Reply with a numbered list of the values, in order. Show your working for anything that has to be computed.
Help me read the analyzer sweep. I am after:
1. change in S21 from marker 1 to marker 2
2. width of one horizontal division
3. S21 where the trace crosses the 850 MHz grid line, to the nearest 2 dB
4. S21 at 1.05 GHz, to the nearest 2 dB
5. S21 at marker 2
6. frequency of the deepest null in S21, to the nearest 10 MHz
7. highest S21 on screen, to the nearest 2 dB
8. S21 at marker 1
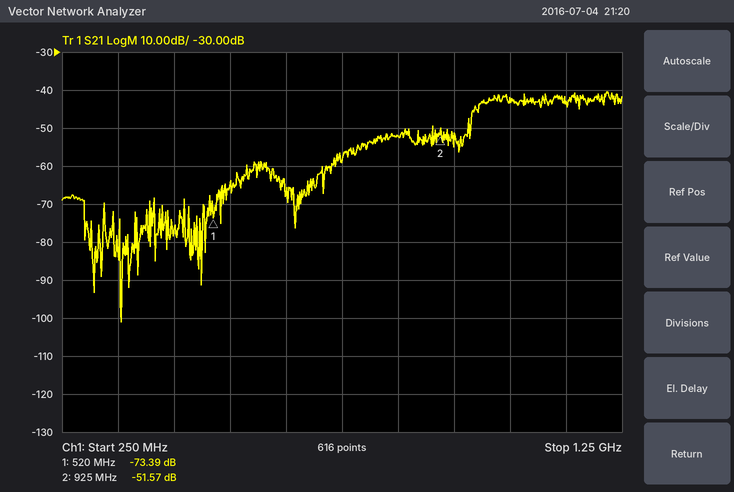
1. -51.57 − (-73.39) = 21.82 dB
2. 100 MHz
3. -52 dB
4. -42 dB
5. -51.57 dB
6. 360 MHz
7. -40 dB
8. -73.39 dB
